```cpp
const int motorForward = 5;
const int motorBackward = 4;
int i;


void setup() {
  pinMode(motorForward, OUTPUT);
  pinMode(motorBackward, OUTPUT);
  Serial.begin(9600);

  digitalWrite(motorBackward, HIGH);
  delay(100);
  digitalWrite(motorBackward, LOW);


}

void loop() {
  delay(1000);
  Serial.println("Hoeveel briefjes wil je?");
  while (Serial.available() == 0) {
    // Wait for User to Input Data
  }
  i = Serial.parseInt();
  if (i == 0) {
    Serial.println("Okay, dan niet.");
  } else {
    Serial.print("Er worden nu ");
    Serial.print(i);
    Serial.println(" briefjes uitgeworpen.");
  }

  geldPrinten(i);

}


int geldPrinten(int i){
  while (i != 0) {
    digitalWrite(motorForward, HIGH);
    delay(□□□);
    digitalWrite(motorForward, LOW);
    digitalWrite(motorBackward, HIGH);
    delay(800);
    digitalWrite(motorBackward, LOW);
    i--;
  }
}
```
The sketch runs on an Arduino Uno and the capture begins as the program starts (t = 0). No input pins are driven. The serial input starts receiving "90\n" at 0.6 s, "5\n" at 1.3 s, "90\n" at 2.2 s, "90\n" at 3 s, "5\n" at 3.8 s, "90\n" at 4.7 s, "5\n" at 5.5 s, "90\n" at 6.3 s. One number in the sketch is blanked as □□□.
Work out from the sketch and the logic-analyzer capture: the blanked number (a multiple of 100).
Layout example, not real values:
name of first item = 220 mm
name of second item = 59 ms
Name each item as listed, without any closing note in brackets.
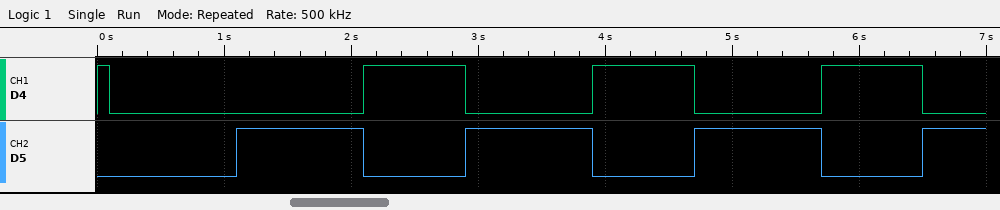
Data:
the blanked number = 1000
